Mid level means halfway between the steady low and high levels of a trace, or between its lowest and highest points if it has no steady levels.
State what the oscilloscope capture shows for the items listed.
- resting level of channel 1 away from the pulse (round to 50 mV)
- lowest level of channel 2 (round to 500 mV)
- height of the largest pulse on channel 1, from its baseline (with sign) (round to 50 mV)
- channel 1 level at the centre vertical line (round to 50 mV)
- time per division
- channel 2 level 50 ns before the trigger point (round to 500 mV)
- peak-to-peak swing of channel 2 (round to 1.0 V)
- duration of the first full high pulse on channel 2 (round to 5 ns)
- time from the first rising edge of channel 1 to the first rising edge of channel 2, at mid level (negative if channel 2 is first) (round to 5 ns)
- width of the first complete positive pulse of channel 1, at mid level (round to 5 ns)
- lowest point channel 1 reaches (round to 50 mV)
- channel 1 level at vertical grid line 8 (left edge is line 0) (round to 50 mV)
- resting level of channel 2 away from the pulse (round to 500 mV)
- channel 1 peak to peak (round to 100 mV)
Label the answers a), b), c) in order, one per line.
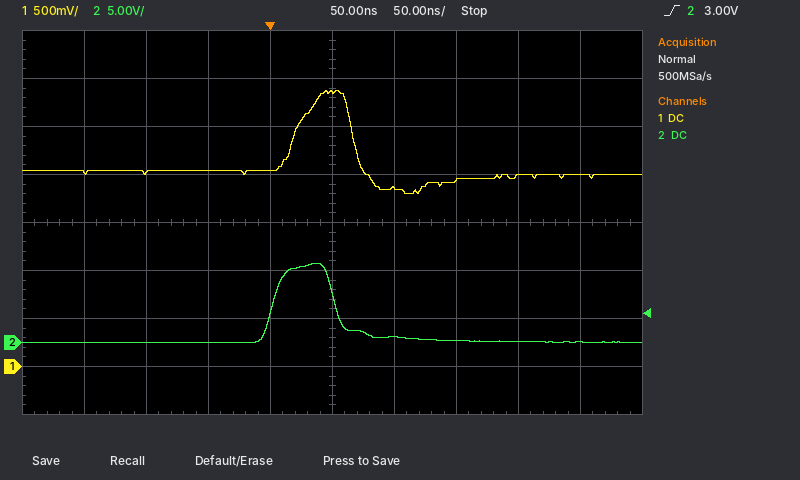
a) 2.05 V
b) 0.0 V
c) +850 mV
d) 2.85 V
e) 50 ns
f) 0.0 V
g) 8.0 V
h) 50 ns
i) -15 ns
j) 50 ns
k) 1.80 V
l) 2.00 V
m) 0.0 V
n) 1.10 V
